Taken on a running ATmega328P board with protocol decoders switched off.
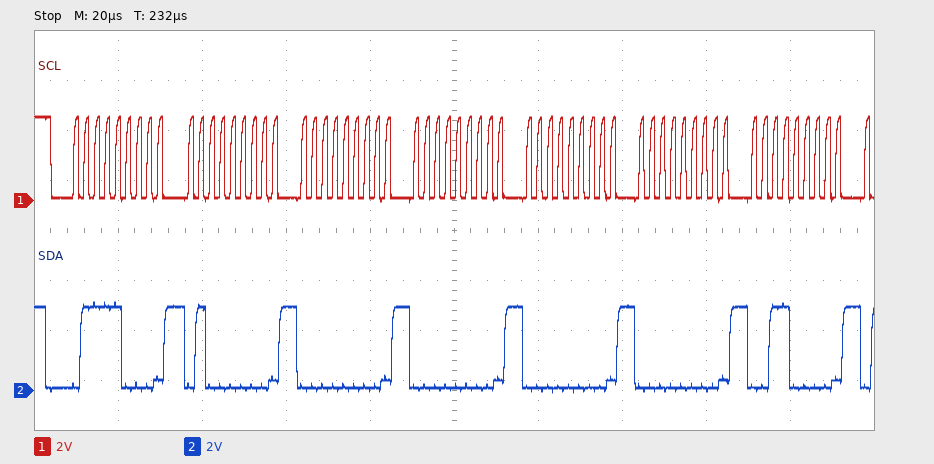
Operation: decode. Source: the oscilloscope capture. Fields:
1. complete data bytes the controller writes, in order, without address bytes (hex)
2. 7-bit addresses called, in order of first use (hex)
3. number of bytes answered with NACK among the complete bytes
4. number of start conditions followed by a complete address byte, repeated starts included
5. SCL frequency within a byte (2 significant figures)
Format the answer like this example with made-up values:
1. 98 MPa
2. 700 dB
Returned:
1. 40 00 00 00 00 30
2. 0x3C
3. 0
4. 1
5. 400 kHz
